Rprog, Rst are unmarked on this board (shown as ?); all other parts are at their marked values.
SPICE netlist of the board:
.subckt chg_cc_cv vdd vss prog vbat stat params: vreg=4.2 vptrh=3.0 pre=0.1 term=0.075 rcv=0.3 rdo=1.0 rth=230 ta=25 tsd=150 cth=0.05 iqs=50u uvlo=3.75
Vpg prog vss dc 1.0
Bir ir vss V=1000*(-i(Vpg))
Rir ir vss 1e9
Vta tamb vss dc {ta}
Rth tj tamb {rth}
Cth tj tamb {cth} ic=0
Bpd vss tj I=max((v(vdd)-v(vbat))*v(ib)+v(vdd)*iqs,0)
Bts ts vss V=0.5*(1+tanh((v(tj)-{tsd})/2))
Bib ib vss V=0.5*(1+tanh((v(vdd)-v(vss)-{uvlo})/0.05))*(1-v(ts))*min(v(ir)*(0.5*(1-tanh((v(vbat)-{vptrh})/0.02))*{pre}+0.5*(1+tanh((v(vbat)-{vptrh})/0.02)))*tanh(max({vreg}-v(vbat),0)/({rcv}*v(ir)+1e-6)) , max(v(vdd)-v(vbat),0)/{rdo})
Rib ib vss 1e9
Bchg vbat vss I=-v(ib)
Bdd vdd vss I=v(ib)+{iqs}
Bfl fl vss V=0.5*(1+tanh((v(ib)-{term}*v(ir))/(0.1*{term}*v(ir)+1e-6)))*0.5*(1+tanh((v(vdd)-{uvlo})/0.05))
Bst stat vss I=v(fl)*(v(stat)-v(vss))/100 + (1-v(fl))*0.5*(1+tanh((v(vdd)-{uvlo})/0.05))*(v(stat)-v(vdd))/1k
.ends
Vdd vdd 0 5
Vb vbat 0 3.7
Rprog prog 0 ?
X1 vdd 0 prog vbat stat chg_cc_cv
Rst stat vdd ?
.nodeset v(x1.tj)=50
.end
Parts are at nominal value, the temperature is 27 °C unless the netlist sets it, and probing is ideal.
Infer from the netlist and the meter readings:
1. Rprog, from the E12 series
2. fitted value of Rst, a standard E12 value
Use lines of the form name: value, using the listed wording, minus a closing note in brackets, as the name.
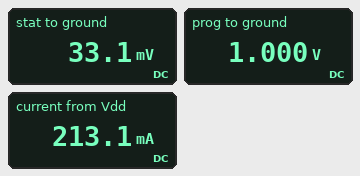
Rprog, from the E12 series: 4.7 kΩ
fitted value of Rst, a standard E12 value: 15 kΩ
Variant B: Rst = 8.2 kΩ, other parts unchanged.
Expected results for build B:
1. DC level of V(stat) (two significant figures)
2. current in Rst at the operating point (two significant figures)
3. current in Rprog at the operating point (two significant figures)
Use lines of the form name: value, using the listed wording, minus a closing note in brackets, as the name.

DC level of V(stat): 60 mV
current in Rst at the operating point: 600 µA
current in Rprog at the operating point: 210 µA
